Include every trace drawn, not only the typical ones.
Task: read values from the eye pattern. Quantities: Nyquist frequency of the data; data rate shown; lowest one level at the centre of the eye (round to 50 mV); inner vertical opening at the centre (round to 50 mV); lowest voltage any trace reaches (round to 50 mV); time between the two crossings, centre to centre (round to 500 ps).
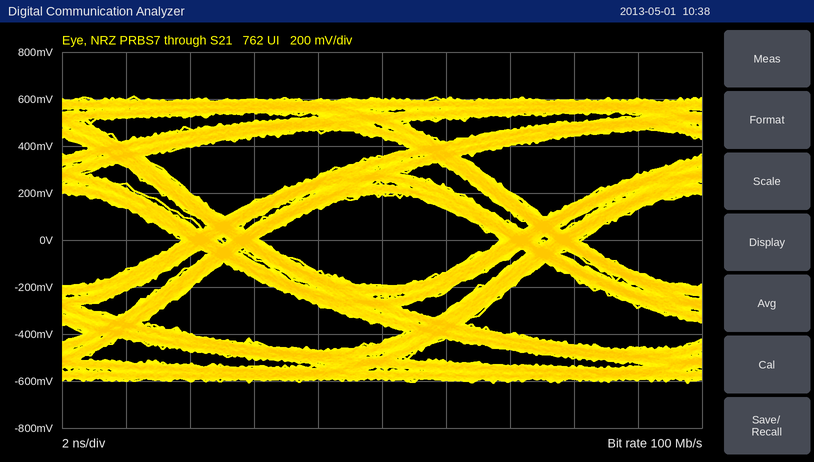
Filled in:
50 MHz
100 Mb/s
200 mV
400 mV
-600 mV
10.0 ns
